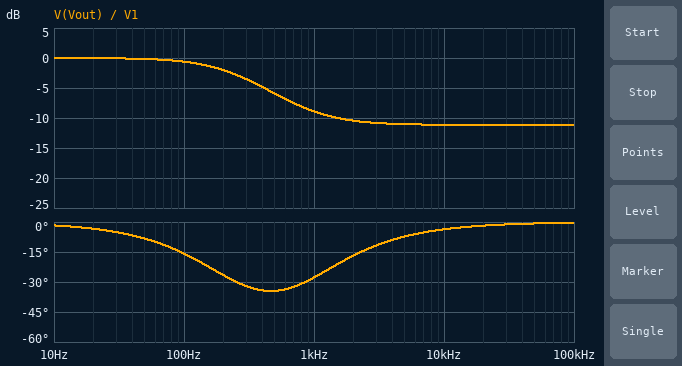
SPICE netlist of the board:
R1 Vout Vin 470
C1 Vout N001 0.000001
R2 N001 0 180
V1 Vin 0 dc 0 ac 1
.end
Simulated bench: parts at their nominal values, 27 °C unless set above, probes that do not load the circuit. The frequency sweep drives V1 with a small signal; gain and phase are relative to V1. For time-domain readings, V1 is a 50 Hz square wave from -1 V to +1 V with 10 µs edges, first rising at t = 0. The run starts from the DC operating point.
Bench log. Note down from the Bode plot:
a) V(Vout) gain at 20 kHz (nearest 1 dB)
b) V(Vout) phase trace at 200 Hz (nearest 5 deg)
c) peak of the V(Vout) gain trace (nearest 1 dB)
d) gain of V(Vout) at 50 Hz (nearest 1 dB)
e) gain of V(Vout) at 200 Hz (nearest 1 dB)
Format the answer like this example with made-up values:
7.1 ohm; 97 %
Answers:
-11 dB; -25 deg; 0 dB; 0 dB; -2 dB
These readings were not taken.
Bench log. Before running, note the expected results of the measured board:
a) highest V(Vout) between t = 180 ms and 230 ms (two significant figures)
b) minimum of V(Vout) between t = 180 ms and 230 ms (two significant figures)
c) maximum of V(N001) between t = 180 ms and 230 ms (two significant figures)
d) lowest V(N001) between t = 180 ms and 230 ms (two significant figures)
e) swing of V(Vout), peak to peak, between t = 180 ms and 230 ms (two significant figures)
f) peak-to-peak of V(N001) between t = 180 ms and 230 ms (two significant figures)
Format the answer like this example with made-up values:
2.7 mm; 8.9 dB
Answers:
1.0 V; -1.0 V; 550 mV; -550 mV; 2.0 V; 1.1 V
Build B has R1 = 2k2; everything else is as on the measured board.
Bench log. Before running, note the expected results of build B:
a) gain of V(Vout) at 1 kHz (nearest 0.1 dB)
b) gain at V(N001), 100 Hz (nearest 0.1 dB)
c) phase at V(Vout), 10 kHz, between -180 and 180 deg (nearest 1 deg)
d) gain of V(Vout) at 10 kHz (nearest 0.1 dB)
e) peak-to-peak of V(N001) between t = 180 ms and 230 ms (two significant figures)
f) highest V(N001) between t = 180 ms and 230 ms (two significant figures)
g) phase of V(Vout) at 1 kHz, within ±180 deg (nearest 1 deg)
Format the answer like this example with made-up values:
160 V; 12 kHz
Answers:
-19.9 dB; -24.0 dB; -5 deg; -22.4 dB; 300 mV; 150 mV; -38 deg
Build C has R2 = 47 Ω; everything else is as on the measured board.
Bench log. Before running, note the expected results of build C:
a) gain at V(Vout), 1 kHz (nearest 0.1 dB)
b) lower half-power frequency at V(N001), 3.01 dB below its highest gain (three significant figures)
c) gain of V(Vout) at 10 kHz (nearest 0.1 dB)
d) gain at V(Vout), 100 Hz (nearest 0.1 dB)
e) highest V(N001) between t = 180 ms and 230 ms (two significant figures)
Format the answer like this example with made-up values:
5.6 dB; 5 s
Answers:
-10.3 dB; 308 Hz; -20.4 dB; -0.4 dB; 180 mV
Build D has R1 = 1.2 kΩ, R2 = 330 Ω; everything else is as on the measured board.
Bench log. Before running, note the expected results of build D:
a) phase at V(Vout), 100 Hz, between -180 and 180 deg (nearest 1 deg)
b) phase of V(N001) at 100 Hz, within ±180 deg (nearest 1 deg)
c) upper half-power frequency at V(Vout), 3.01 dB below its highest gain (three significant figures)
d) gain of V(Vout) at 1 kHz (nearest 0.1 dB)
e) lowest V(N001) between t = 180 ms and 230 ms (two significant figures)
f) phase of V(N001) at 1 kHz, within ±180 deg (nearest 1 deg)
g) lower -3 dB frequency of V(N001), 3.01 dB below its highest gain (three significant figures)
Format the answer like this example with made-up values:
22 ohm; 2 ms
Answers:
-32 deg; 46 deg; 109 Hz; -12.5 dB; -430 mV; 6 deg; 104 Hz
